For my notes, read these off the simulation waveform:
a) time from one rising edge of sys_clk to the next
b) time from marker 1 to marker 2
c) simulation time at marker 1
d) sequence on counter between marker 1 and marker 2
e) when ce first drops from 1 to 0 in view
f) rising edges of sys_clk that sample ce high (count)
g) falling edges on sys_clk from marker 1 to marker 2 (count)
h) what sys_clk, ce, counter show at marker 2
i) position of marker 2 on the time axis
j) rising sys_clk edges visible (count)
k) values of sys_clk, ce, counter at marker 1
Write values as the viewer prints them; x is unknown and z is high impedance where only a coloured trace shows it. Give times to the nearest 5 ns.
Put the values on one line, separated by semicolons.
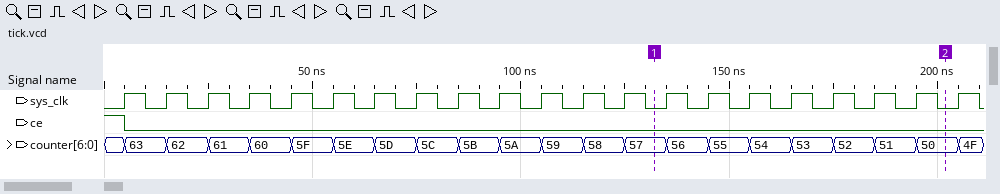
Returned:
10 ns; 70 ns; 130 ns; 57, 56, 55, 54, 53, 52, 51, 50; 5 ns; 1; 7; sys_clk=0, ce=0, counter=50; 200 ns; 21; sys_clk=0, ce=0, counter=57
